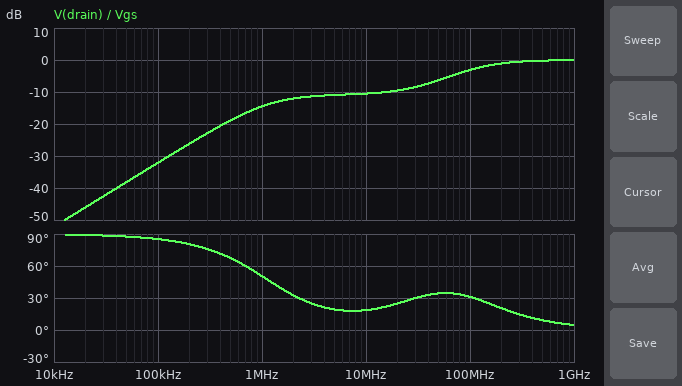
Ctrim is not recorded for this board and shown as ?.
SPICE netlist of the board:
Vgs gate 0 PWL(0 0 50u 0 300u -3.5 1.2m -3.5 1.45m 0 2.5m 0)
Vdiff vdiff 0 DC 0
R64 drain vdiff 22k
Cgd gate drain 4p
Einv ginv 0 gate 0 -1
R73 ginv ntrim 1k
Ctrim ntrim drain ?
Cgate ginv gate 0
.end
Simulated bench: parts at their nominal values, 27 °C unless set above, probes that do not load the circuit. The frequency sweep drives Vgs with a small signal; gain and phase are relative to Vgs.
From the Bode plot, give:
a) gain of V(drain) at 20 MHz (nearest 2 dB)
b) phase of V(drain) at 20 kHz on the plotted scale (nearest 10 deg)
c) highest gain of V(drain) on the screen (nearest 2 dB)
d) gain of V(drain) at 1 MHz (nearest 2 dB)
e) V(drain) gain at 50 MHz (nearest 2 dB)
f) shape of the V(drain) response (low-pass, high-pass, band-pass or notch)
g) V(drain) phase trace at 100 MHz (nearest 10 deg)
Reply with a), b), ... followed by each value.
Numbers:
a) -10 dB
b) 90 deg
c) 0 dB
d) -14 dB
e) -6 dB
f) high-pass
g) 30 deg
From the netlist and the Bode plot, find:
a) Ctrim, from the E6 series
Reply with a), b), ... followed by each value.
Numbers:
a) 2.2 pF
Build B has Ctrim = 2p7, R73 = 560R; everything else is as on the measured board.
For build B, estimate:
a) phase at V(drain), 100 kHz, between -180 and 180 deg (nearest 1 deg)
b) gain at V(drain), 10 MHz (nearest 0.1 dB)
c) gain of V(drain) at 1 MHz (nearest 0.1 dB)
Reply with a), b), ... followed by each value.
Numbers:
a) 85 deg
b) -14.0 dB
c) -17.6 dB
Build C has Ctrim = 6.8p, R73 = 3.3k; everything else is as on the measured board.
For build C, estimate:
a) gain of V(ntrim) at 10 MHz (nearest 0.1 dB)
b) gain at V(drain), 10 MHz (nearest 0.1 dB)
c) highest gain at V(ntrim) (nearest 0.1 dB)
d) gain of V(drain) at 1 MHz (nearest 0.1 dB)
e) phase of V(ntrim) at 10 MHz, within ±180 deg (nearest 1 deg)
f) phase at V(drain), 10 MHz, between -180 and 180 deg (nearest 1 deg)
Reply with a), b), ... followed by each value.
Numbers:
a) -0.2 dB
b) -6.2 dB
c) 0 dB
d) -13.5 dB
e) 127 deg
f) 94 deg
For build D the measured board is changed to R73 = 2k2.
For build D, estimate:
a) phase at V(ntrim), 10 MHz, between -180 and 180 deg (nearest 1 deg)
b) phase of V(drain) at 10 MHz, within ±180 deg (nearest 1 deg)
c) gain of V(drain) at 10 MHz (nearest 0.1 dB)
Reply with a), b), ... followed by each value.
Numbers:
a) 158 deg
b) 30 deg
c) -9.4 dB
